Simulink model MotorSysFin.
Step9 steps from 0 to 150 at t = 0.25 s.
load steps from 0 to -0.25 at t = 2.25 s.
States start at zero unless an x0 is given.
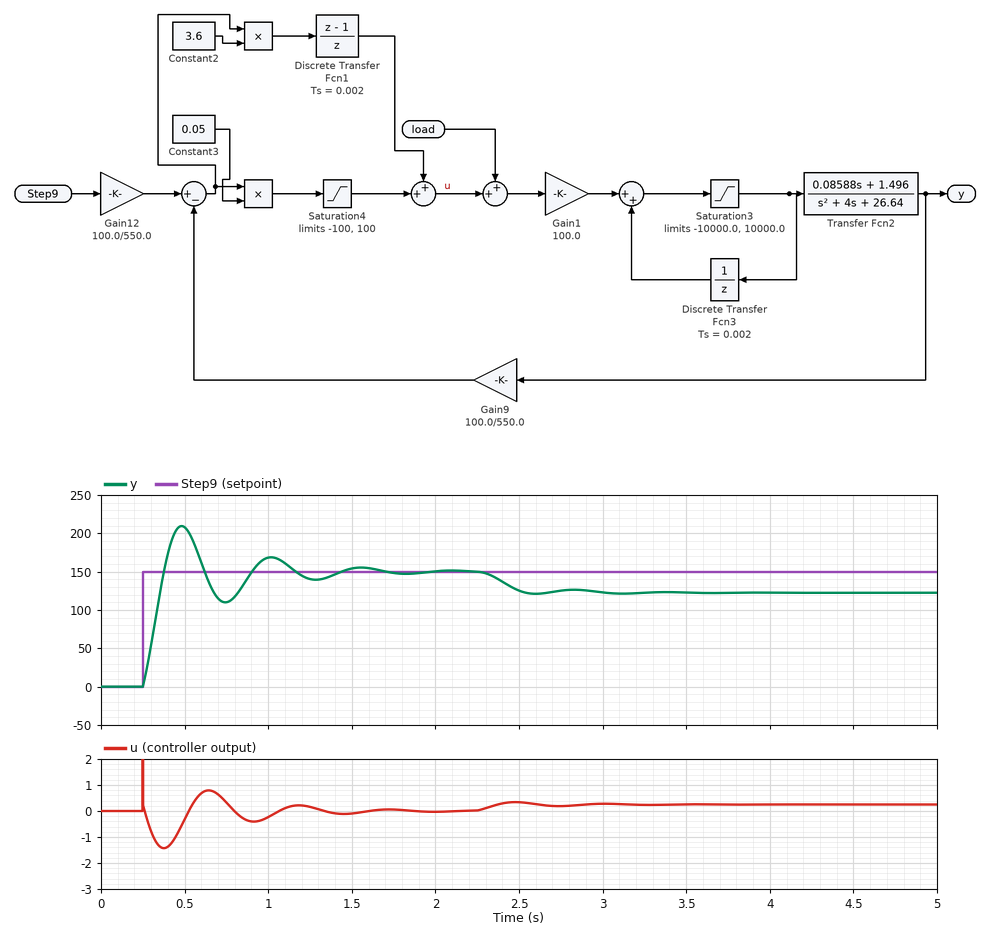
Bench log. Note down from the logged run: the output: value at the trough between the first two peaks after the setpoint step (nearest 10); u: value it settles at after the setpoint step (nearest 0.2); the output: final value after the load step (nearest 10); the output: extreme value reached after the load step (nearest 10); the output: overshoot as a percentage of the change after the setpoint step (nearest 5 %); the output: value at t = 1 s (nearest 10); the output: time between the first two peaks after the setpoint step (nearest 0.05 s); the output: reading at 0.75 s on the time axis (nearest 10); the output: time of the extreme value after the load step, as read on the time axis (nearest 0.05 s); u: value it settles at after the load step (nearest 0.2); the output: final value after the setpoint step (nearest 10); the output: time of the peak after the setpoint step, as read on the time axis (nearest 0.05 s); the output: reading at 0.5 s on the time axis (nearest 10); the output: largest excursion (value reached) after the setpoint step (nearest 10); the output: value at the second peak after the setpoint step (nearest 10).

110
0.0
120
120
40 %
170
0.55 s
110
2.60 s
0.2
150
0.50 s
210
210
170
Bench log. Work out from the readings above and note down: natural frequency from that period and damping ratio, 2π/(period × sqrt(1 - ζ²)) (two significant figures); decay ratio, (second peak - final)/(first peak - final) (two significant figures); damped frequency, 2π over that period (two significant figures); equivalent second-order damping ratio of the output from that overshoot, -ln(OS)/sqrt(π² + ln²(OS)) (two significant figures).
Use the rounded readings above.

12 rad/s
0.33
11 rad/s
0.28
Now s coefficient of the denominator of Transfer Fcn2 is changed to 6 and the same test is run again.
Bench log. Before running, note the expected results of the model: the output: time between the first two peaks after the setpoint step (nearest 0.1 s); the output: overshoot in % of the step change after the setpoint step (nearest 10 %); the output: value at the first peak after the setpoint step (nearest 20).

0.6 s
30 %
200
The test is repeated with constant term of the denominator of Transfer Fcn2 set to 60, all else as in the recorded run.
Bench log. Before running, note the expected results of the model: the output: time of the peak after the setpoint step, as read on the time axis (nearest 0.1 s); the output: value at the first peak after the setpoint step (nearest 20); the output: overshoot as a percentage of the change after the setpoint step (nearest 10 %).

0.5 s
180
20 %
